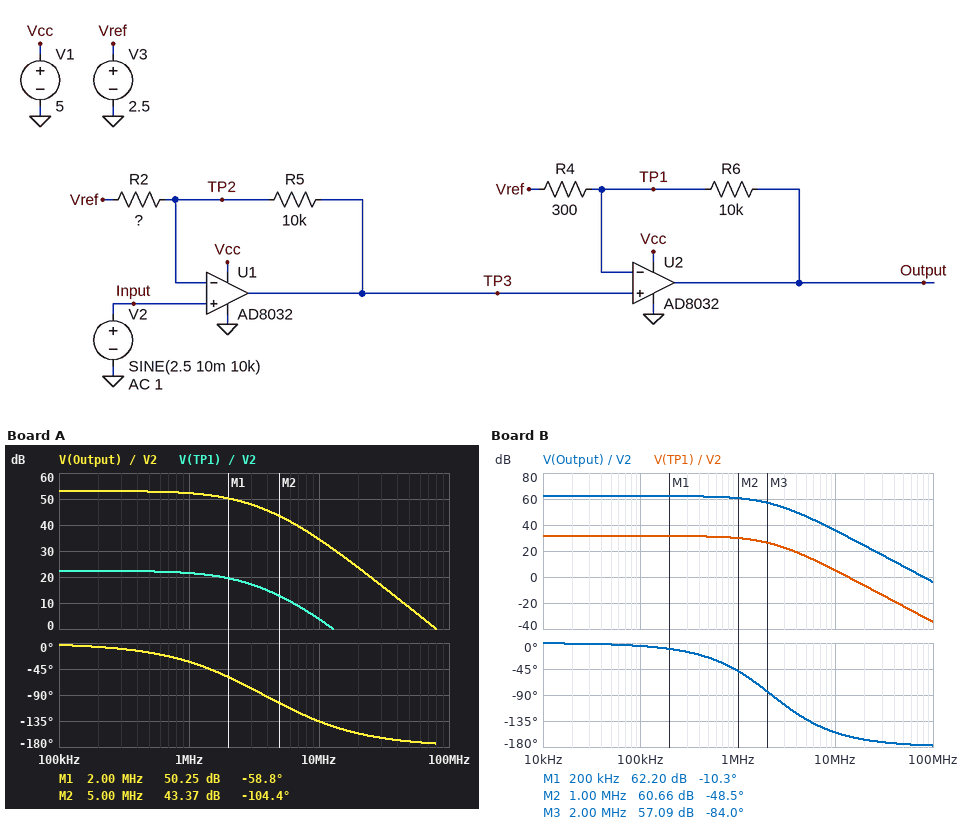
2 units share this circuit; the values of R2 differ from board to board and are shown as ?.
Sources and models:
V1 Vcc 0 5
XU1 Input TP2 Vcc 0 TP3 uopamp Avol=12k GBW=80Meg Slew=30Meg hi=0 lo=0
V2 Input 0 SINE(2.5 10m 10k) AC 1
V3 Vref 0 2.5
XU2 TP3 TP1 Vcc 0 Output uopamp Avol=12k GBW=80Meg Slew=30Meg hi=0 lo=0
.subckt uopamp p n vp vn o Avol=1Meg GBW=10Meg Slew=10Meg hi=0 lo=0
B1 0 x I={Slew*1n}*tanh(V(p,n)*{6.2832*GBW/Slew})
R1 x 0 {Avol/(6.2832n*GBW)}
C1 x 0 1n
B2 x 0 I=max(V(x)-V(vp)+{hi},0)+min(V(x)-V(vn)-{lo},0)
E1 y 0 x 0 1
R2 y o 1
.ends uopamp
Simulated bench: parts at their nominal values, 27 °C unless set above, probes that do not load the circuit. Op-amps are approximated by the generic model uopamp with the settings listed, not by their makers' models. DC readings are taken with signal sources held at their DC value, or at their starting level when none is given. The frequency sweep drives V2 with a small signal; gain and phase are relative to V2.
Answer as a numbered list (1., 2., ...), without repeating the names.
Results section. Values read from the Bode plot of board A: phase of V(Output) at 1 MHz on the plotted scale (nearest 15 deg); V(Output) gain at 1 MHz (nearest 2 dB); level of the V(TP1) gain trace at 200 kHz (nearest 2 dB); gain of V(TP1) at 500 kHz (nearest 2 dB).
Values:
1. -30 deg
2. 52 dB
3. 22 dB
4. 22 dB
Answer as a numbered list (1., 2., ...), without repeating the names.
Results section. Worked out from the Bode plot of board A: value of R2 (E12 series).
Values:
1. 820 Ω
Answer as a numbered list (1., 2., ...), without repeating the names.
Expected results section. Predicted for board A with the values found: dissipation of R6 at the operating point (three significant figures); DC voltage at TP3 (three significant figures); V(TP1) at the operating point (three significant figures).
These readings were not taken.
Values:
1. 964 nW
2. 2.50 V
3. 2.50 V
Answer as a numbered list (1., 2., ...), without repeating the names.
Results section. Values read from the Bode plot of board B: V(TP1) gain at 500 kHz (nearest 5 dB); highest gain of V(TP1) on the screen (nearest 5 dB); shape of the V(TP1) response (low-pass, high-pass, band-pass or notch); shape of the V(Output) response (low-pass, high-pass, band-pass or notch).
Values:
1. 30 dB
2. 30 dB
3. low-pass
4. low-pass
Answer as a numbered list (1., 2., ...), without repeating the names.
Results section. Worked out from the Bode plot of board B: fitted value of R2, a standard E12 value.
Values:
1. 270 Ω
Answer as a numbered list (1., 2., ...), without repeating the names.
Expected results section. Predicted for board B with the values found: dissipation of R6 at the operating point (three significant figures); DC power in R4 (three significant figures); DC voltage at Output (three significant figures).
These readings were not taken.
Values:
1. 7.26 µW
2. 218 nW
3. 2.22 V
